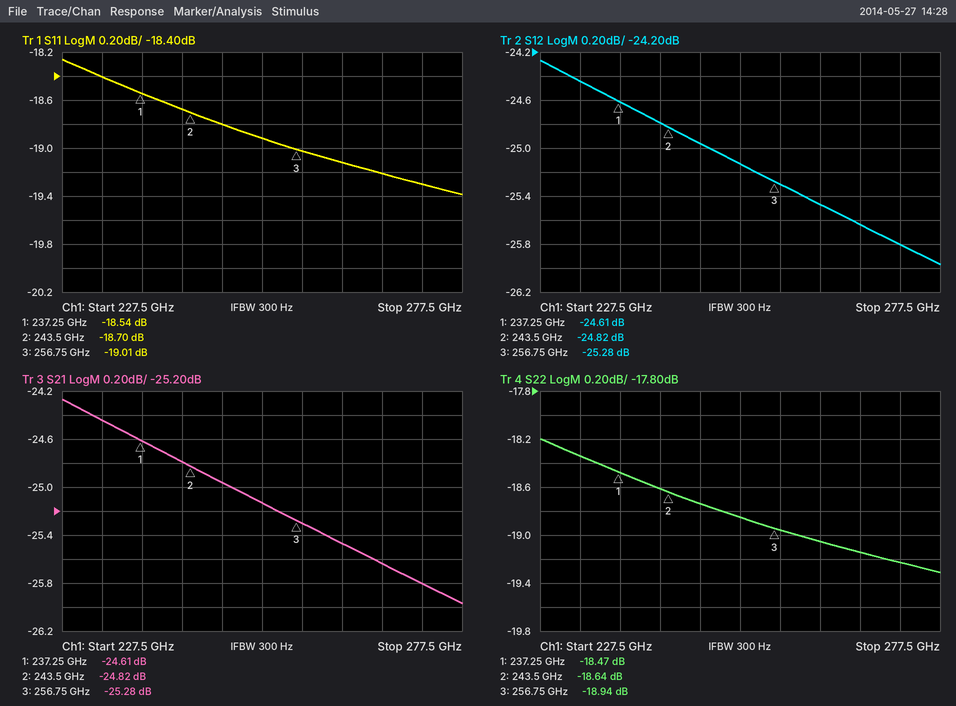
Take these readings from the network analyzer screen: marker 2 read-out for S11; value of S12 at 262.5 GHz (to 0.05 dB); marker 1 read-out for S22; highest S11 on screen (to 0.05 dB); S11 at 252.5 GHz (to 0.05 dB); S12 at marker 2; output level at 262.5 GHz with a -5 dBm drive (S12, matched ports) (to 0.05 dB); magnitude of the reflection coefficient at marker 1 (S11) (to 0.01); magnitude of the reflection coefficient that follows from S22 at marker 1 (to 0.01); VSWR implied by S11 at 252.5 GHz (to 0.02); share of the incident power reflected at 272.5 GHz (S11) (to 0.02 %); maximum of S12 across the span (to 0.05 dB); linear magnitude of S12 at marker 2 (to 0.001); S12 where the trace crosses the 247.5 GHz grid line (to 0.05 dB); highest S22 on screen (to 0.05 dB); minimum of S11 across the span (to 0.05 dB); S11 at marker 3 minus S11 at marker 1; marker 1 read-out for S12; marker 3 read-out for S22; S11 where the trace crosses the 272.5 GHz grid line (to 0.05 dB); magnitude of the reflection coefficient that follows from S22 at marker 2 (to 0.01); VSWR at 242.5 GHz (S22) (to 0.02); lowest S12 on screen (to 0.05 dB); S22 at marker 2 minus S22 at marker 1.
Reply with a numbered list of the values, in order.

1. -18.70 dB
2. -25.45 dB
3. -18.47 dB
4. -18.25 dB
5. -18.90 dB
6. -24.82 dB
7. -30.45 dBm
8. 0.12
9. 0.12
10. 1.26
11. 1.18 %
12. -24.25 dB
13. 0.057
14. -24.95 dB
15. -18.20 dB
16. -19.40 dB
17. -0.47 dB
18. -24.61 dB
19. -18.94 dB
20. -19.30 dB
21. 0.12
22. 1.26
23. -25.95 dB
24. -0.17 dB
